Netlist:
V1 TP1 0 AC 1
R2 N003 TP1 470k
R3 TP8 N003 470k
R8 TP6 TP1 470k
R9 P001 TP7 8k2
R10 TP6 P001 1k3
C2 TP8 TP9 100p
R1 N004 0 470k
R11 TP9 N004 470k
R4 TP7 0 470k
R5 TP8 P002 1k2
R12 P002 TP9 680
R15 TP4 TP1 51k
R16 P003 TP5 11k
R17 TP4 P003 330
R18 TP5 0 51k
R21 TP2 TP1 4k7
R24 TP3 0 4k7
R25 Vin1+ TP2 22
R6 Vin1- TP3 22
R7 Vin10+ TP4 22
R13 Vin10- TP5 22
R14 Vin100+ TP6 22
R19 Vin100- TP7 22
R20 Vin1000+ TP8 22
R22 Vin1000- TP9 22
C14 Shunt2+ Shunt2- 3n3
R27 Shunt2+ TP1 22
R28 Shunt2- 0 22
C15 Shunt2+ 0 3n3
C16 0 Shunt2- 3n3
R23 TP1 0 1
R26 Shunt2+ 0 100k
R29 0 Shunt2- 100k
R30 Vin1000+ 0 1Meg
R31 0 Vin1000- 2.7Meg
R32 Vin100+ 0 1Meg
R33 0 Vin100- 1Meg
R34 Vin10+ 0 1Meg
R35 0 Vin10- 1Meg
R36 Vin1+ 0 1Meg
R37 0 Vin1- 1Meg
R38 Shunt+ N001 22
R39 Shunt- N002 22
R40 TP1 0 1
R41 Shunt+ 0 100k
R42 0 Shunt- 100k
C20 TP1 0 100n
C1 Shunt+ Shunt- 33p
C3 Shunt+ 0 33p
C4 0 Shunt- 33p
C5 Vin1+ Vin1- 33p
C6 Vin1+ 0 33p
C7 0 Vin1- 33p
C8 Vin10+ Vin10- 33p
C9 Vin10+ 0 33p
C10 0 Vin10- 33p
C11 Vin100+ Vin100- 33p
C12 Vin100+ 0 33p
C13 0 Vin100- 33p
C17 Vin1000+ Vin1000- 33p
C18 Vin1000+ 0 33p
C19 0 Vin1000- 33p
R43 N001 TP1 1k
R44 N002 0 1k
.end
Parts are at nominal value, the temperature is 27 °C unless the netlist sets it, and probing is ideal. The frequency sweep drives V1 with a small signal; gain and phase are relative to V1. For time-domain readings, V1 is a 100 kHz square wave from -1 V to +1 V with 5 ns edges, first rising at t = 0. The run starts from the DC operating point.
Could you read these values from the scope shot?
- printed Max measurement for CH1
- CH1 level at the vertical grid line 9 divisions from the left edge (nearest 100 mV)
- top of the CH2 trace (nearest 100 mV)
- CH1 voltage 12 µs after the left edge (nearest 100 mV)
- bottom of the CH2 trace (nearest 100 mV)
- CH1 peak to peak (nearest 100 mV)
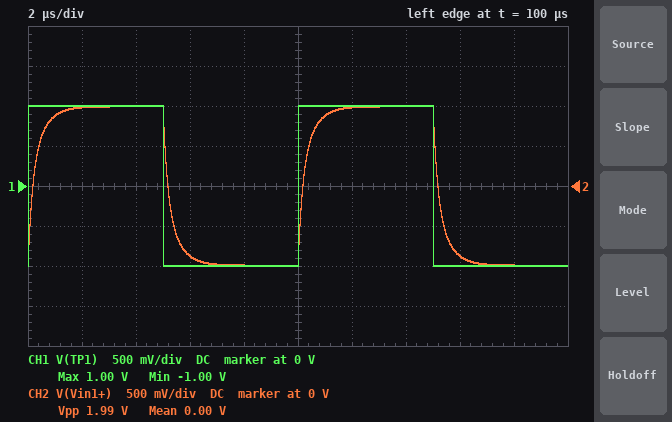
1.00 V
-1.0 V
1.0 V
1.0 V
-1.0 V
2.0 V
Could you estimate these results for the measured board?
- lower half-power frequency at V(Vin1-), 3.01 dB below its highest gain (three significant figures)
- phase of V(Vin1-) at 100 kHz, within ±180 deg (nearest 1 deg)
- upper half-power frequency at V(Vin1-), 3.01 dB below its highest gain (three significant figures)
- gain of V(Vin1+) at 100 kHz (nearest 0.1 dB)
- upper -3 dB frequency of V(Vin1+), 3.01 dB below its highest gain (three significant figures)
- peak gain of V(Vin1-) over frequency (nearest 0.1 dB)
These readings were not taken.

221 kHz
68 deg
1.59 MHz
-0.3 dB
503 kHz
-12.1 dB
